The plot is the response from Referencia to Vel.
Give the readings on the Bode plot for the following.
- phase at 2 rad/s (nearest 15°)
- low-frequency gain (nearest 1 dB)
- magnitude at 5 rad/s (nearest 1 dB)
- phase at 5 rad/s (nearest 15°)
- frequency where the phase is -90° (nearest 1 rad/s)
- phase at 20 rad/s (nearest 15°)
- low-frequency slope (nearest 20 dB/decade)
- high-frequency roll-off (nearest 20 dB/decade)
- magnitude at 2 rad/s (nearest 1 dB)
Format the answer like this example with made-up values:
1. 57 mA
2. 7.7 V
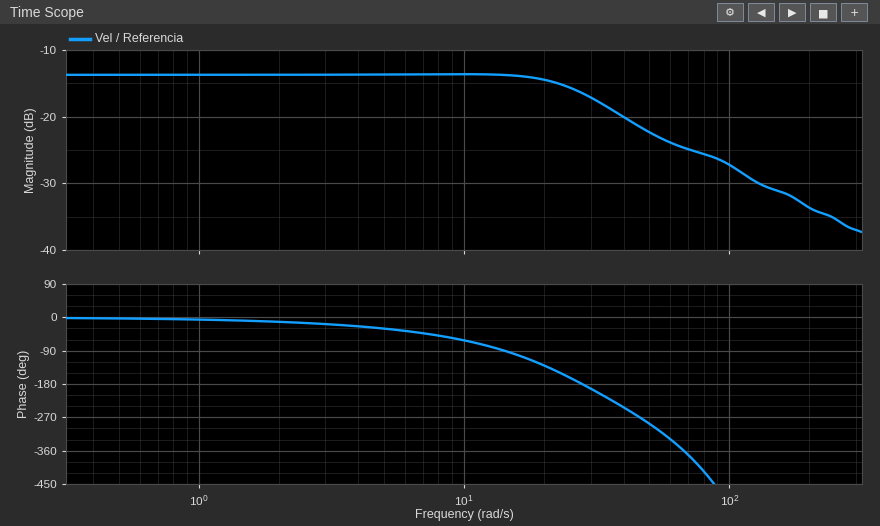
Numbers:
1. -15°
2. -14 dB
3. -14 dB
4. -30°
5. 14 rad/s
6. -135°
7. 0 dB/decade
8. -20 dB/decade
9. -14 dB
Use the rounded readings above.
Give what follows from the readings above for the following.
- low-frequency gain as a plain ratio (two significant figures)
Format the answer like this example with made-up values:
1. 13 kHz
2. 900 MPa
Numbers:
1. 0.20
